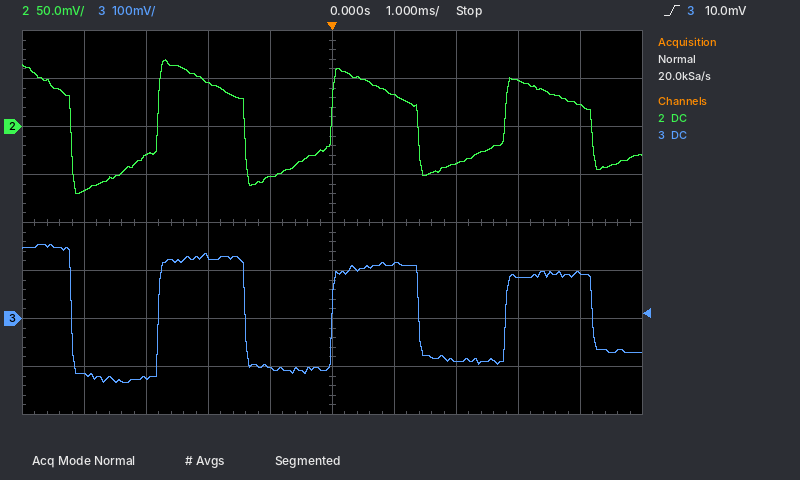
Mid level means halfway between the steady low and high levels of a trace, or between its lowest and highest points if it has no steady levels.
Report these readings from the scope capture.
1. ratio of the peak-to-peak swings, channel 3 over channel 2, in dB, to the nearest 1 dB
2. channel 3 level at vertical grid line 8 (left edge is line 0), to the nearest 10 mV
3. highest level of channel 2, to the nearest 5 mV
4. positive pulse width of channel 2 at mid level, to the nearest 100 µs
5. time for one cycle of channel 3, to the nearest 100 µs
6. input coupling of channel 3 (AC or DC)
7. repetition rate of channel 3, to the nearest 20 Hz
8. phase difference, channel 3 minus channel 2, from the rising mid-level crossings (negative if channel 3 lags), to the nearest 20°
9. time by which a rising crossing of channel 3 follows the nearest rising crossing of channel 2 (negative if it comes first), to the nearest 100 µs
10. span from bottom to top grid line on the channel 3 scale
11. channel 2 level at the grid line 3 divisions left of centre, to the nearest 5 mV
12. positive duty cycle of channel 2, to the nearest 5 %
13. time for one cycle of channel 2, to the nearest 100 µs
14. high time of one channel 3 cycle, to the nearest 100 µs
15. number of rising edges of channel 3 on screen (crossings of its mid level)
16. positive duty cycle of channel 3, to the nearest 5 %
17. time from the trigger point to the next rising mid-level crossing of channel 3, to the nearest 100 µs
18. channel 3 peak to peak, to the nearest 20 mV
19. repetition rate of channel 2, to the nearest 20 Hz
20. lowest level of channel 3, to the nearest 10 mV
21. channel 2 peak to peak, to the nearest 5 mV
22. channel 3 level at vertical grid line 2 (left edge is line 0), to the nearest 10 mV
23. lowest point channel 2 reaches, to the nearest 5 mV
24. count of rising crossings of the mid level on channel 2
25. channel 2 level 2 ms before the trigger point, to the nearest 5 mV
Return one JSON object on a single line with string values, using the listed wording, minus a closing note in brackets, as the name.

{"ratio of the peak-to-peak swings, channel 3 over channel 2, in dB, to the nearest 1 dB": "6 dB", "channel 3 level at vertical grid line 8 (left edge is line 0), to the nearest 10 mV": "90 mV", "highest level of channel 2, to the nearest 5 mV": "70 mV", "positive pulse width of channel 2 at mid level, to the nearest 100 µs": "1.4 ms", "time for one cycle of channel 3, to the nearest 100 µs": "2.8 ms", "input coupling of channel 3": "DC", "repetition rate of channel 3, to the nearest 20 Hz": "360 Hz", "phase difference, channel 3 minus channel 2, from the rising mid-level crossings (negative if channel 3 lags), to the nearest 20°": "0°", "time by which a rising crossing of channel 3 follows the nearest rising crossing of channel 2 (negative if it comes first), to the nearest 100 µs": "0.0 ms", "span from bottom to top grid line on the channel 3 scale": "800 mV", "channel 2 level at the grid line 3 divisions left of centre, to the nearest 5 mV": "-30 mV", "positive duty cycle of channel 2, to the nearest 5 %": "50 %", "time for one cycle of channel 2, to the nearest 100 µs": "2.8 ms", "high time of one channel 3 cycle, to the nearest 100 µs": "1.4 ms", "number of rising edges of channel 3 on screen": "3", "positive duty cycle of channel 3, to the nearest 5 %": "50 %", "time from the trigger point to the next rising mid-level crossing of channel 3, to the nearest 100 µs": "2.8 ms", "channel 3 peak to peak, to the nearest 20 mV": "280 mV", "repetition rate of channel 2, to the nearest 20 Hz": "360 Hz", "lowest level of channel 3, to the nearest 10 mV": "-130 mV", "channel 2 peak to peak, to the nearest 5 mV": "140 mV", "channel 3 level at vertical grid line 2 (left edge is line 0), to the nearest 10 mV": "-120 mV", "lowest point channel 2 reaches, to the nearest 5 mV": "-70 mV", "count of rising crossings of the mid level on channel 2": "3", "channel 2 level 2 ms before the trigger point, to the nearest 5 mV": "45 mV"}
